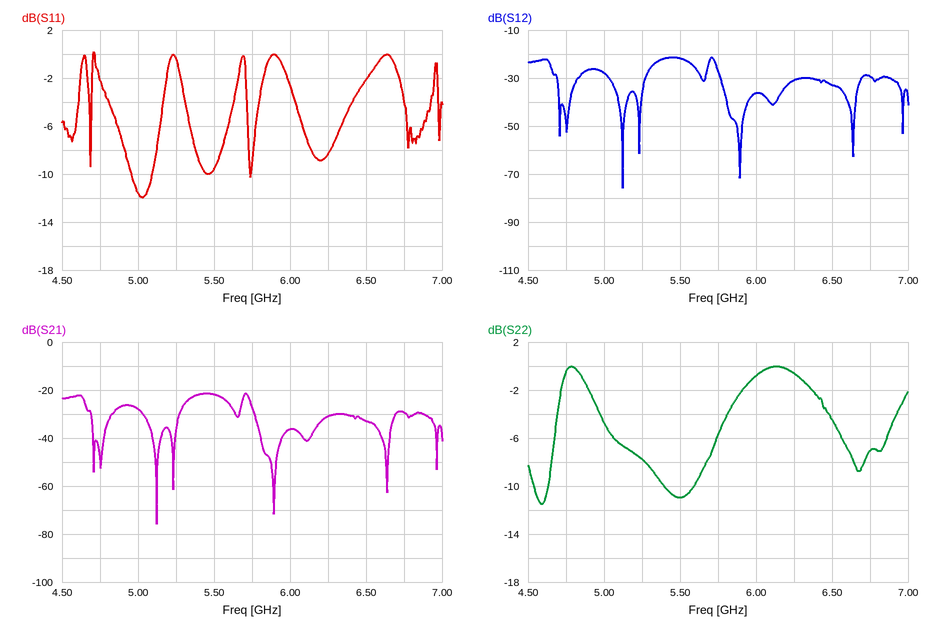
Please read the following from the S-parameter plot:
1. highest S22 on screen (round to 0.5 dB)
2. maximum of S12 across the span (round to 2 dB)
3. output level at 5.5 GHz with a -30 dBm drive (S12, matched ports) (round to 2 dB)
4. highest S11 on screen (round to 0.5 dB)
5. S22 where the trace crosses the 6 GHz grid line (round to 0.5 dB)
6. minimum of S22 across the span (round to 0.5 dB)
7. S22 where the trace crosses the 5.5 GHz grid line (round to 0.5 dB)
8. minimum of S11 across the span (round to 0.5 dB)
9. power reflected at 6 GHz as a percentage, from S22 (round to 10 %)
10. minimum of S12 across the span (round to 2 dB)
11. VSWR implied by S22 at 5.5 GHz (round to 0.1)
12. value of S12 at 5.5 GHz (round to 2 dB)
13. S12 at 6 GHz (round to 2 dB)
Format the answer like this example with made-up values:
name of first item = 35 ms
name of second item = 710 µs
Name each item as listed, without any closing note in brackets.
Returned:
highest S22 on screen = 0.0 dB
maximum of S12 across the span = -22 dB
output level at 5.5 GHz with a -30 dBm drive (S12, matched ports) = -52 dBm
highest S11 on screen = 0.0 dB
S22 where the trace crosses the 6 GHz grid line = -1.0 dB
minimum of S22 across the span = -11.5 dB
S22 where the trace crosses the 5.5 GHz grid line = -11.0 dB
minimum of S11 across the span = -12.0 dB
power reflected at 6 GHz as a percentage, from S22 = 80 %
minimum of S12 across the span = -76 dB
VSWR implied by S22 at 5.5 GHz = 1.8
value of S12 at 5.5 GHz = -22 dB
S12 at 6 GHz = -36 dB
